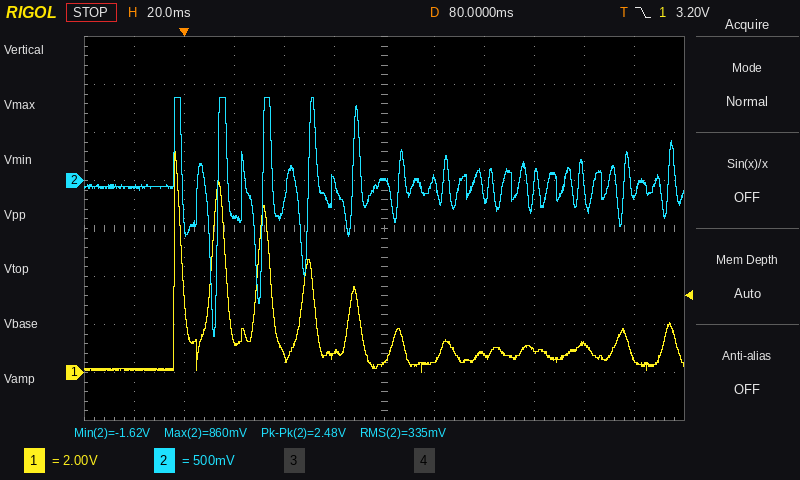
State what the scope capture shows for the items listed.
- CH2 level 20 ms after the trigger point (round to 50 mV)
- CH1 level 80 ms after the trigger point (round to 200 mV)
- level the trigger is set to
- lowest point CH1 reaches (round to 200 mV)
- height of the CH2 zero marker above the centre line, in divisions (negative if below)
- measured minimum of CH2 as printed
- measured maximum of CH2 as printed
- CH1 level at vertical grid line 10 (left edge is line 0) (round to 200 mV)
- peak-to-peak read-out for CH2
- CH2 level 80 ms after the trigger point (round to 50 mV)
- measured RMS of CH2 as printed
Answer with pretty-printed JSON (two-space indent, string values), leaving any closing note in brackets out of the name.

{
  "CH2 level 20 ms after the trigger point": "-350 mV",
  "CH1 level 80 ms after the trigger point": "400 mV",
  "level the trigger is set to": "3.20 V",
  "lowest point CH1 reaches": "0.0 V",
  "height of the CH2 zero marker above the centre line, in divisions": "+1.0 div",
  "measured minimum of CH2 as printed": "-1.62 V",
  "measured maximum of CH2 as printed": "860 mV",
  "CH1 level at vertical grid line 10 (left edge is line 0)": "1.2 V",
  "peak-to-peak read-out for CH2": "2.48 V",
  "CH2 level 80 ms after the trigger point": "0 mV",
  "measured RMS of CH2 as printed": "335 mV"
}
